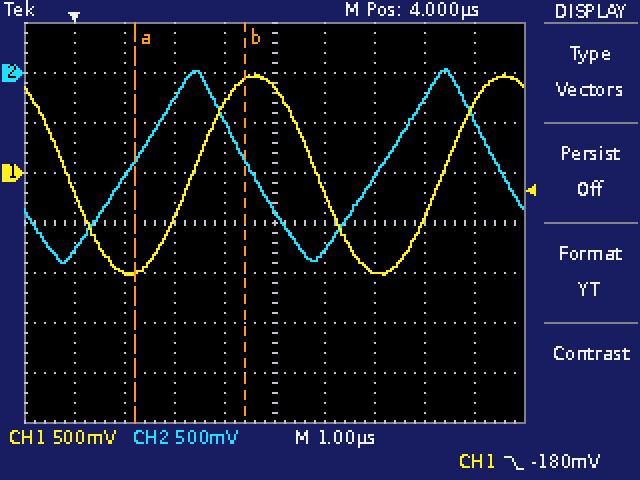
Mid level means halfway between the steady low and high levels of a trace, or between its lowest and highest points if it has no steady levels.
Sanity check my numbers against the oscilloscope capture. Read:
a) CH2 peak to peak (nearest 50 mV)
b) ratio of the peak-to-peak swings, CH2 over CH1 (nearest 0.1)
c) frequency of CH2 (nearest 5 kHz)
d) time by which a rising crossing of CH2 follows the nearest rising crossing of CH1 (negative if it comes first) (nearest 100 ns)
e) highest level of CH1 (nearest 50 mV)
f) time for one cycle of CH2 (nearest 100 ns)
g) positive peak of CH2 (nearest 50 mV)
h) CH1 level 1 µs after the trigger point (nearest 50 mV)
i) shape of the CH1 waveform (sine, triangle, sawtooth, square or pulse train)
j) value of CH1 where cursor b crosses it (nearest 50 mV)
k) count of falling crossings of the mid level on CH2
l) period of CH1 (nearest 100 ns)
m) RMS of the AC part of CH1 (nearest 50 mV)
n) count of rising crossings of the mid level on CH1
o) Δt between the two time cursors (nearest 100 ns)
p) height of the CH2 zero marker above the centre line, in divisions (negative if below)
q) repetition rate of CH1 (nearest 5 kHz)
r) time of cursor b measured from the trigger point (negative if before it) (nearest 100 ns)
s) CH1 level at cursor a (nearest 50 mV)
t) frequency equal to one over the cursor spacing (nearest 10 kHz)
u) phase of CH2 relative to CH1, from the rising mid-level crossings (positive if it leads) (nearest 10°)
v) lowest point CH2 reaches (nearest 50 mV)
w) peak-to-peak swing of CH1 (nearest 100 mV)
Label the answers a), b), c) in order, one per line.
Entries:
a) 1.95 V
b) 1.0
c) 200 kHz
d) -1.2 µs
e) 1.00 V
f) 5.0 µs
g) 50 mV
h) -1.00 V
i) sine
j) 950 mV
k) 2
l) 5.0 µs
m) 700 mV
n) 2
o) 2.2 µs
p) +3.0 div
q) 200 kHz
r) +3.4 µs
s) -1.00 V
t) 450 kHz
u) +90°
v) -1.90 V
w) 2.00 V
